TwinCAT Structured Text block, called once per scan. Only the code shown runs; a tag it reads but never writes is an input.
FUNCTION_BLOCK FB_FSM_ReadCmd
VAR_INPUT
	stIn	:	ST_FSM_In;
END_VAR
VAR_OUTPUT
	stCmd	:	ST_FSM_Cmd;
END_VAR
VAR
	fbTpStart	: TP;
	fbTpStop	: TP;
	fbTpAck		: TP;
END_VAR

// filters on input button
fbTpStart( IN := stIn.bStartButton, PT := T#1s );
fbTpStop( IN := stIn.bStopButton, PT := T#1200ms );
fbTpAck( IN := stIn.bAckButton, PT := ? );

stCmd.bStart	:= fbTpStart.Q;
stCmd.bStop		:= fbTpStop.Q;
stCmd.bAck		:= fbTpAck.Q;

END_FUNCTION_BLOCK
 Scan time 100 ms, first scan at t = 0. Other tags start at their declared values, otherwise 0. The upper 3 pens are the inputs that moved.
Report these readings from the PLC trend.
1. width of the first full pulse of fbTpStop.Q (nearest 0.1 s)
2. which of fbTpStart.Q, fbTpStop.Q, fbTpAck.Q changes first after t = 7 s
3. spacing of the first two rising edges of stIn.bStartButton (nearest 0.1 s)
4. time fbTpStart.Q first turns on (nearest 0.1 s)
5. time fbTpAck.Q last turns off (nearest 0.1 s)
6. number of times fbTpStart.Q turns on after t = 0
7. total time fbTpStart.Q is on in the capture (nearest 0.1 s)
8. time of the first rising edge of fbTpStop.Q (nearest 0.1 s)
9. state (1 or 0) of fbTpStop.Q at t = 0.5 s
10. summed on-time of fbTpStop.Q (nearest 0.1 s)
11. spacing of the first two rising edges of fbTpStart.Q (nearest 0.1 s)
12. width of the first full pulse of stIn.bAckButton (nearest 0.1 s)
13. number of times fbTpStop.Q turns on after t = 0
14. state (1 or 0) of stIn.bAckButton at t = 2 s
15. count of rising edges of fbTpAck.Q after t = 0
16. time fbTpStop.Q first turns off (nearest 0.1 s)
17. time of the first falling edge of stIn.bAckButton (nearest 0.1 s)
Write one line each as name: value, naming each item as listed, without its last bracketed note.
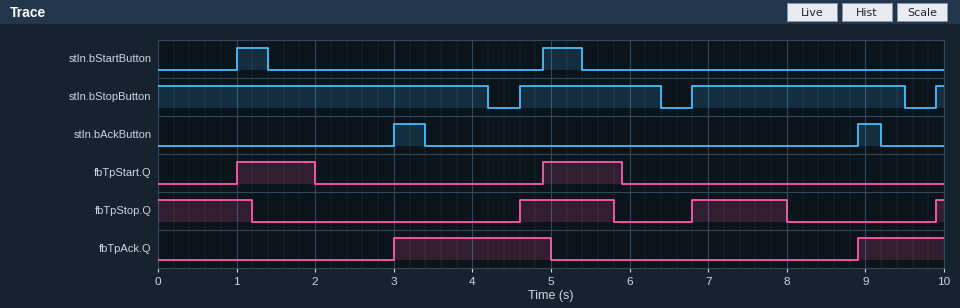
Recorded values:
width of the first full pulse of fbTpStop.Q: 1.2 s
which of fbTpStart.Q, fbTpStop.Q, fbTpAck.Q changes first after t = 7 s: fbTpStop.Q
spacing of the first two rising edges of stIn.bStartButton: 3.9 s
time fbTpStart.Q first turns on: 1.0 s
time fbTpAck.Q last turns off: 5.0 s
number of times fbTpStart.Q turns on after t = 0: 2
total time fbTpStart.Q is on in the capture: 2.0 s
time of the first rising edge of fbTpStop.Q: 4.6 s
state (1 or 0) of fbTpStop.Q at t = 0.5 s: 1
summed on-time of fbTpStop.Q: 3.7 s
spacing of the first two rising edges of fbTpStart.Q: 3.9 s
width of the first full pulse of stIn.bAckButton: 0.4 s
number of times fbTpStop.Q turns on after t = 0: 3
state (1 or 0) of stIn.bAckButton at t = 2 s: 0
count of rising edges of fbTpAck.Q after t = 0: 2
time fbTpStop.Q first turns off: 1.2 s
time of the first falling edge of stIn.bAckButton: 3.4 s
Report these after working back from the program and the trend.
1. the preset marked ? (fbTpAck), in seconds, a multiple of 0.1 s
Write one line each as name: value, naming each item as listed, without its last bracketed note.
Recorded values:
the preset marked ? (fbTpAck), in seconds, a multiple of 0.1 s: 2.0 s
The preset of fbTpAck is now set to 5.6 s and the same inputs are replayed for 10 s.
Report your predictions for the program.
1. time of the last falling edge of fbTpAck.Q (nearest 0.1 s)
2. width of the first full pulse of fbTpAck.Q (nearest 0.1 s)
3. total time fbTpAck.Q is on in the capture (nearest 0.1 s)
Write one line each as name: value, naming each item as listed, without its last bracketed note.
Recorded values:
time of the last falling edge of fbTpAck.Q: 8.6 s
width of the first full pulse of fbTpAck.Q: 5.6 s
total time fbTpAck.Q is on in the capture: 6.7 s
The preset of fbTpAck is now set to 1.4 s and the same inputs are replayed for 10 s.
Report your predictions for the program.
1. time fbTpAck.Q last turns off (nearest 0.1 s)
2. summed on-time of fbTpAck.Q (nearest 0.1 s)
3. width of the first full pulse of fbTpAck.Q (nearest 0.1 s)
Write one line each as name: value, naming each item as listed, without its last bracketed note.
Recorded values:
time fbTpAck.Q last turns off: 4.4 s
summed on-time of fbTpAck.Q: 2.5 s
width of the first full pulse of fbTpAck.Q: 1.4 s
